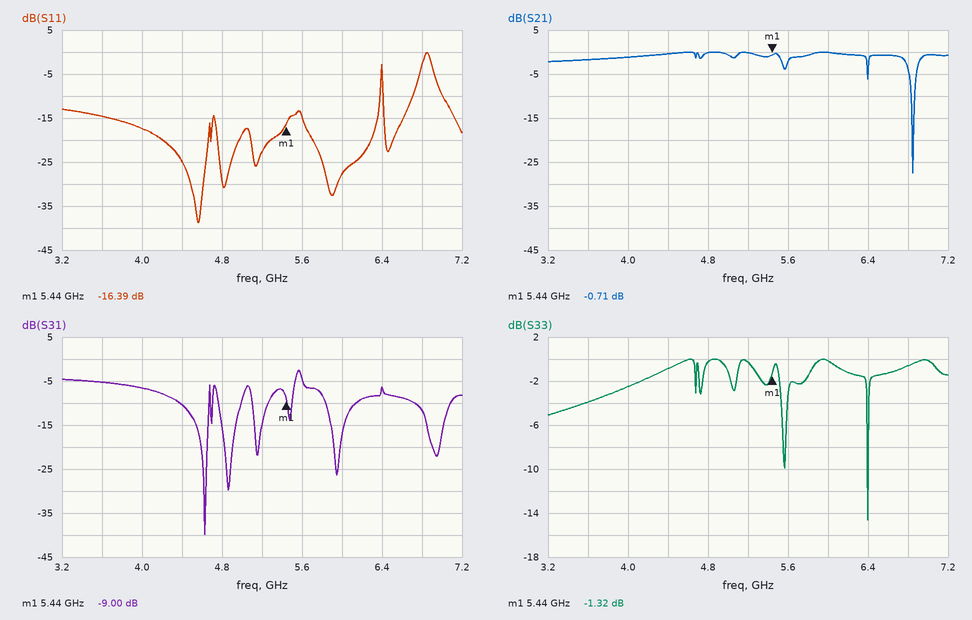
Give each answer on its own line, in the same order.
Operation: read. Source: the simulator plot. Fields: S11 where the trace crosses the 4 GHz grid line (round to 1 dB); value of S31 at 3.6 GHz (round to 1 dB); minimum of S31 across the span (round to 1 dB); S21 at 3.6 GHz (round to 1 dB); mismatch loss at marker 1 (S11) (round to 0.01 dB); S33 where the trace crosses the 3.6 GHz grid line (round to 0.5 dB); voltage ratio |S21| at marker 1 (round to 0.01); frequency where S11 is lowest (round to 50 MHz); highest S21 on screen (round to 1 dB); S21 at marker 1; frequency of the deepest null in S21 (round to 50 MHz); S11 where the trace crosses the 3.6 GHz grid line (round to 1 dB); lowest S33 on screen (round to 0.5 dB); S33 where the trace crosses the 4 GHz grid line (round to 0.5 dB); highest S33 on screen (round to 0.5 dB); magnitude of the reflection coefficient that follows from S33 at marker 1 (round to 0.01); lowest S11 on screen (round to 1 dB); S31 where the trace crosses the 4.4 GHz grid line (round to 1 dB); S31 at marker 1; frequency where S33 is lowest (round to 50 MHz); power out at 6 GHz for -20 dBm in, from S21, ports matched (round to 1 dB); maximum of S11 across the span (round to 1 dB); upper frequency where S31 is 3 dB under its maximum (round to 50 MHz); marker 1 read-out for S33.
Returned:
-17 dB
-5 dB
-40 dB
-2 dB
0.10 dB
-4.0 dB
0.92
4.55 GHz
0 dB
-0.71 dB
6.85 GHz
-15 dB
-14.5 dB
-2.5 dB
0.0 dB
0.86
-39 dB
-10 dB
-9.00 dB
6.40 GHz
-20 dBm
0 dB
5.60 GHz
-1.32 dB
